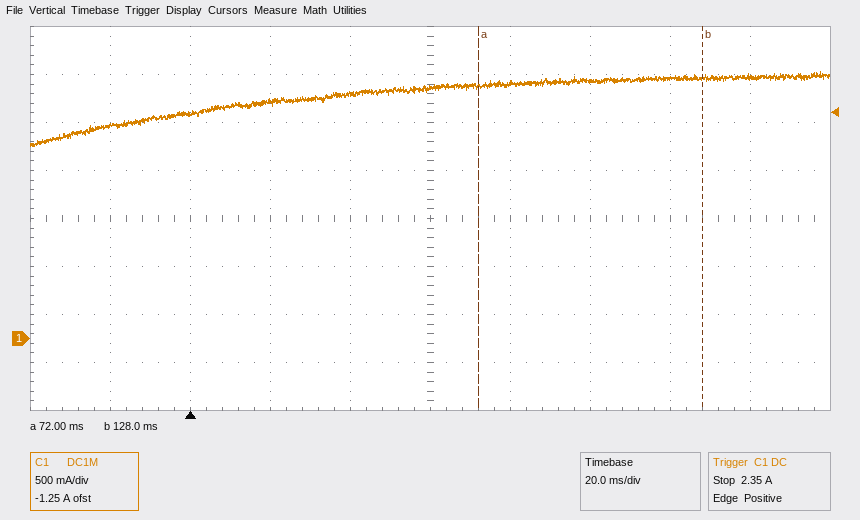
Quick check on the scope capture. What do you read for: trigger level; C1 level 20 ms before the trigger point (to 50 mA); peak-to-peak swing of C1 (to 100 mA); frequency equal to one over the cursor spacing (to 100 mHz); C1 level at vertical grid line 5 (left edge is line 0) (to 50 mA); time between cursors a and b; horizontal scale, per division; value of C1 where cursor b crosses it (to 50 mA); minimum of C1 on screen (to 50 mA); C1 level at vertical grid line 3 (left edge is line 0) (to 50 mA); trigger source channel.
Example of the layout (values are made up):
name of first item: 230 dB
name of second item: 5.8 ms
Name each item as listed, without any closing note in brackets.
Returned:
trigger level: 2.35 A
C1 level 20 ms before the trigger point: 2.20 A
peak-to-peak swing of C1: 800 mA
frequency equal to one over the cursor spacing: 17.9 Hz
C1 level at vertical grid line 5 (left edge is line 0): 2.60 A
time between cursors a and b: 56 ms
horizontal scale, per division: 20 ms
value of C1 where cursor b crosses it: 2.70 A
minimum of C1 on screen: 2.00 A
C1 level at vertical grid line 3 (left edge is line 0): 2.45 A
trigger source channel: C1
